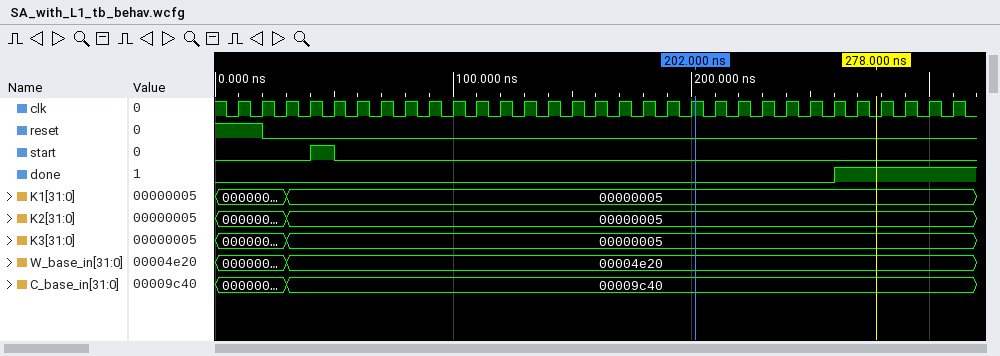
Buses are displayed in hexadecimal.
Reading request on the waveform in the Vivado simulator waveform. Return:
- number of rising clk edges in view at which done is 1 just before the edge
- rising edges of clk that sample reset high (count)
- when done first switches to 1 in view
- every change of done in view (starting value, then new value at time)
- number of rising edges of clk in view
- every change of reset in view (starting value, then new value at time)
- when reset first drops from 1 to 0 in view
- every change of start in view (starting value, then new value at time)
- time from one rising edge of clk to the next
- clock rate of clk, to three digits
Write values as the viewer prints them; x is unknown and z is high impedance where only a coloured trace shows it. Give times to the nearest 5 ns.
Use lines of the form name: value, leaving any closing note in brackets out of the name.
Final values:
number of rising clk edges in view at which done is 1 just before the edge: 5
rising edges of clk that sample reset high: 2
when done first switches to 1 in view: 260 ns
every change of done in view: 0, 1 at 260 ns
number of rising edges of clk in view: 31
every change of reset in view: 1, 0 at 20 ns
when reset first drops from 1 to 0 in view: 20 ns
every change of start in view: 0, 1 at 40 ns, 0 at 50 ns
time from one rising edge of clk to the next: 10 ns
clock rate of clk, to three digits: 100 MHz
